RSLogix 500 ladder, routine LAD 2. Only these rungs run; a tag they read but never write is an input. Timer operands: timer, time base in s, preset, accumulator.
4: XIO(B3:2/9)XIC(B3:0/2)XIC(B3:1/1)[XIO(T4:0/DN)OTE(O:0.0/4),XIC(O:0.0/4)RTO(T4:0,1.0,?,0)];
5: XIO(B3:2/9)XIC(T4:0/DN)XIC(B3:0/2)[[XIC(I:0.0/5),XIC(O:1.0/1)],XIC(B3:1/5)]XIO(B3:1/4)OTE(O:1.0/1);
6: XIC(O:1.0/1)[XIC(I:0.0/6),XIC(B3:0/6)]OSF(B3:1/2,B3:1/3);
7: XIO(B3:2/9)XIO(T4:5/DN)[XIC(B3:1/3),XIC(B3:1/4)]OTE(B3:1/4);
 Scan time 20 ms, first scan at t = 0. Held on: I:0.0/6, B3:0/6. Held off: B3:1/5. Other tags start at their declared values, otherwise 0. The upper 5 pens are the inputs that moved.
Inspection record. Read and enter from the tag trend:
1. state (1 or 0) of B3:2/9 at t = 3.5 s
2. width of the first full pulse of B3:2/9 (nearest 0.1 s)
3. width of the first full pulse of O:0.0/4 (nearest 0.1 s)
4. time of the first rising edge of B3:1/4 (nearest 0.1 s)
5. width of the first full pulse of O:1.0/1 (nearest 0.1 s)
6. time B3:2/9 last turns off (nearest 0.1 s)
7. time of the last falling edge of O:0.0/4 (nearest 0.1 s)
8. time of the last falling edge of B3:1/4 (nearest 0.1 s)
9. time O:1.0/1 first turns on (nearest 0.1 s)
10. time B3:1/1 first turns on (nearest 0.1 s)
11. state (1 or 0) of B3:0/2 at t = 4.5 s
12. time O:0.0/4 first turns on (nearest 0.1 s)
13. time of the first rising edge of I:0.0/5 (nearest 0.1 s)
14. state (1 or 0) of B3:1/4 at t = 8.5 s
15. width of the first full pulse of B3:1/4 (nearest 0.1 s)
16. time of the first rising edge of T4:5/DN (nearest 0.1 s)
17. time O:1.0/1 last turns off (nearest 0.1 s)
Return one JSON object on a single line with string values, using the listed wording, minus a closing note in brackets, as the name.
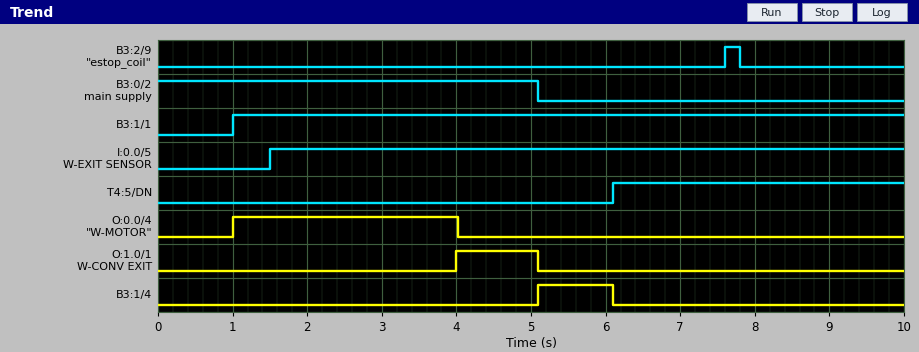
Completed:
{"state (1 or 0) of B3:2/9 at t = 3.5 s": "0", "width of the first full pulse of B3:2/9": "0.2 s", "width of the first full pulse of O:0.0/4": "3.0 s", "time of the first rising edge of B3:1/4": "5.1 s", "width of the first full pulse of O:1.0/1": "1.1 s", "time B3:2/9 last turns off": "7.8 s", "time of the last falling edge of O:0.0/4": "4.0 s", "time of the last falling edge of B3:1/4": "6.1 s", "time O:1.0/1 first turns on": "4.0 s", "time B3:1/1 first turns on": "1.0 s", "state (1 or 0) of B3:0/2 at t = 4.5 s": "1", "time O:0.0/4 first turns on": "1.0 s", "time of the first rising edge of I:0.0/5": "1.5 s", "state (1 or 0) of B3:1/4 at t = 8.5 s": "0", "width of the first full pulse of B3:1/4": "1.0 s", "time of the first rising edge of T4:5/DN": "6.1 s", "time O:1.0/1 last turns off": "5.1 s"}
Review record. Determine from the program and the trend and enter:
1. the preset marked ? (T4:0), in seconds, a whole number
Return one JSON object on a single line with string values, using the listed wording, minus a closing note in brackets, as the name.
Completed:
{"the preset marked ? (T4:0), in seconds, a whole number": "3 s"}
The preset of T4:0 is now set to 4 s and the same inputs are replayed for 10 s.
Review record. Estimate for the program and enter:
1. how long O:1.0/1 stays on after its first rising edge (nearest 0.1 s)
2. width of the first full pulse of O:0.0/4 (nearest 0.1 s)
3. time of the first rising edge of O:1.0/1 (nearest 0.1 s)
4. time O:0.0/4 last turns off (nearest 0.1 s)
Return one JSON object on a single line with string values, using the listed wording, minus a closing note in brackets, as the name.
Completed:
{"how long O:1.0/1 stays on after its first rising edge": "0.1 s", "width of the first full pulse of O:0.0/4": "4.0 s", "time of the first rising edge of O:1.0/1": "5.0 s", "time O:0.0/4 last turns off": "5.0 s"}
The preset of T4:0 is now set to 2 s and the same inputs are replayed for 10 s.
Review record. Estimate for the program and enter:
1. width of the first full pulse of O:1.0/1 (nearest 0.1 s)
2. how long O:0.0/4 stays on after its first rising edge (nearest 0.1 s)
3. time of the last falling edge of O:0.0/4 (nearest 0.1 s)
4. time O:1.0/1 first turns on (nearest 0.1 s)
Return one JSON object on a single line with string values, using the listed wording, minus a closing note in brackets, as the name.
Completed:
{"width of the first full pulse of O:1.0/1": "2.1 s", "how long O:0.0/4 stays on after its first rising edge": "2.0 s", "time of the last falling edge of O:0.0/4": "3.0 s", "time O:1.0/1 first turns on": "3.0 s"}
